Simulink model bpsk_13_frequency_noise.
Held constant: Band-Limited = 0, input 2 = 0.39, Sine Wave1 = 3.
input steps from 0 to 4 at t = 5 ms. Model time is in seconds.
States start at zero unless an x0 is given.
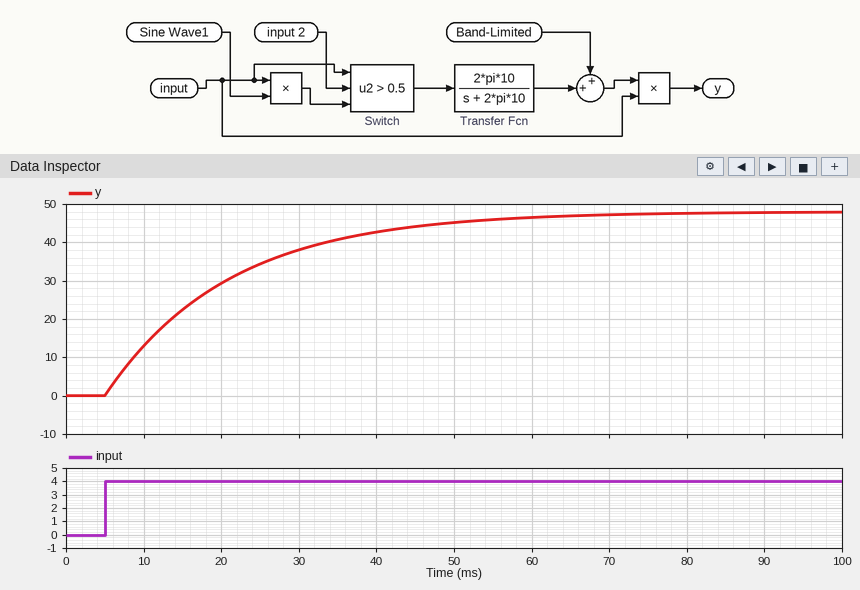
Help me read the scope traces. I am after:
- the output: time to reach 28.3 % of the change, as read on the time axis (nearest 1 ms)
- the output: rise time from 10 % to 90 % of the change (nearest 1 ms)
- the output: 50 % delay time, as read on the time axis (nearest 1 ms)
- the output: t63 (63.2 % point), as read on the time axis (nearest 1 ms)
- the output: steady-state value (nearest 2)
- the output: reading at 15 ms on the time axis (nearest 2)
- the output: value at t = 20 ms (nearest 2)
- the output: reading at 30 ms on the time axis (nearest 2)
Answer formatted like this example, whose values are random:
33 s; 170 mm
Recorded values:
10 ms; 35 ms; 16 ms; 21 ms; 48; 22; 30; 38
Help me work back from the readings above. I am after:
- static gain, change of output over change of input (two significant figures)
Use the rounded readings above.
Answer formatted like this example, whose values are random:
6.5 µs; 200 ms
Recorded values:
12
